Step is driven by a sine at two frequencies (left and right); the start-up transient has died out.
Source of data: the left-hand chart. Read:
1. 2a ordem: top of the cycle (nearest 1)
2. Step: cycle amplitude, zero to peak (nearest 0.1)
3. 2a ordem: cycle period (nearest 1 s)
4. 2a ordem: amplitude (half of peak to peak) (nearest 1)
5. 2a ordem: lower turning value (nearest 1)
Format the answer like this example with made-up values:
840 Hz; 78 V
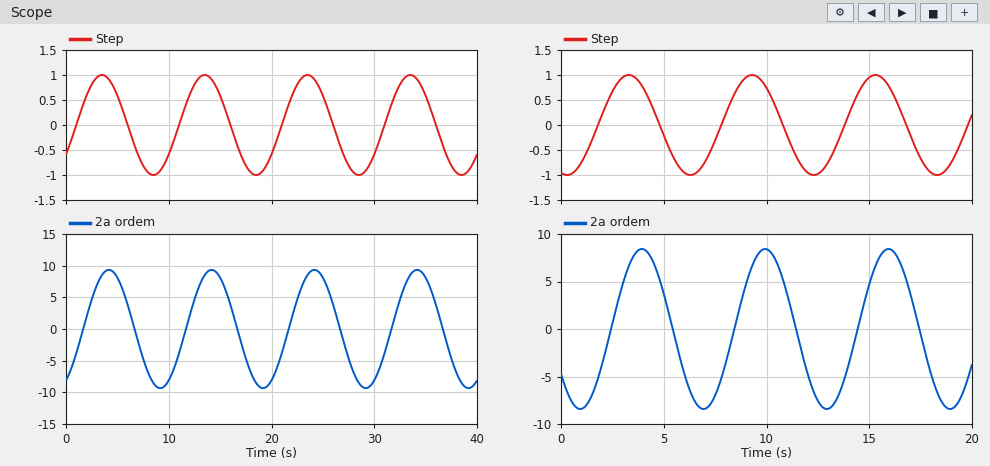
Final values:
9; 1.0; 10 s; 9; -9
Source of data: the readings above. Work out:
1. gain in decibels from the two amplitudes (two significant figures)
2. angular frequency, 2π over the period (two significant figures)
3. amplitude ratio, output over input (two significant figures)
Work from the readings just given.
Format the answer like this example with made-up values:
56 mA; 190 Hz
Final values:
19 dB; 0.63 rad/s; 9.0
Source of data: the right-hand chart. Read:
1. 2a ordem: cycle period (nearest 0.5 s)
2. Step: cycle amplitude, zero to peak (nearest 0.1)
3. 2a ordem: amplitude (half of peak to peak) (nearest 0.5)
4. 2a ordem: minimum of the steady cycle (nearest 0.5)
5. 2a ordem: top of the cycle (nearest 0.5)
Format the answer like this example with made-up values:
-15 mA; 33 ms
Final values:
6.0 s; 1.0; 8.5; -8.5; 8.5
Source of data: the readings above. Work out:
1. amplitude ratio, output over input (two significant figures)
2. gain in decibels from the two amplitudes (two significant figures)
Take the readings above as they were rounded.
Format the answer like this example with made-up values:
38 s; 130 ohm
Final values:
8.5; 19 dB
